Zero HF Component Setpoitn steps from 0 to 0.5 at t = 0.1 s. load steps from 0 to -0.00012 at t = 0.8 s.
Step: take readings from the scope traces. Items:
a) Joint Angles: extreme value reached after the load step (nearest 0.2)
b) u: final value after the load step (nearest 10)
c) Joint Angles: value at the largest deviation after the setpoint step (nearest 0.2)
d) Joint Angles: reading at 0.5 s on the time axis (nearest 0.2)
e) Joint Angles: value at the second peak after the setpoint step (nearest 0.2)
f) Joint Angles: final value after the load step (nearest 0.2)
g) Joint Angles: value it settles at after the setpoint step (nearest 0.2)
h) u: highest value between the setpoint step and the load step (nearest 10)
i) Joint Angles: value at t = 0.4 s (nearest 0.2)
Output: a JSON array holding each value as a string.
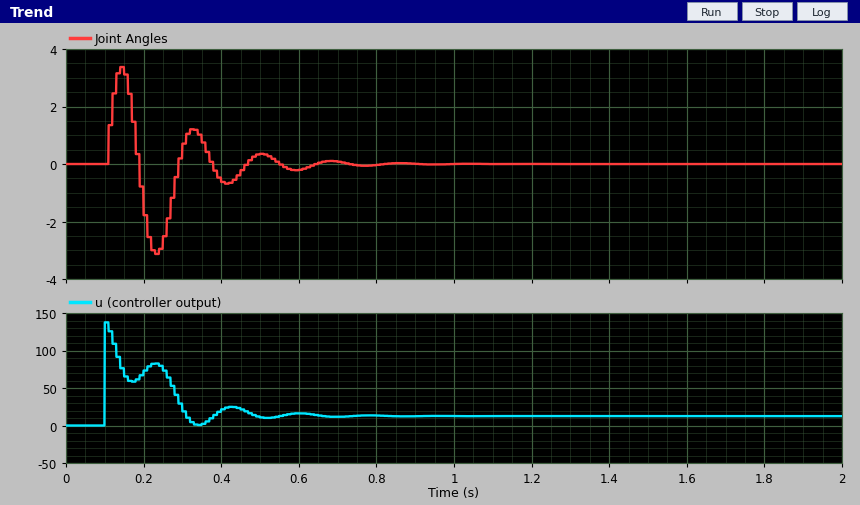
["0.0", "10", "3.4", "0.4", "1.2", "0.0", "0.0", "140", "-0.6"]
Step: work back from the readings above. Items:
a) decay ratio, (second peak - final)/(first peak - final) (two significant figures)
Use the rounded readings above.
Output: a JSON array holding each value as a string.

["0.35"]
